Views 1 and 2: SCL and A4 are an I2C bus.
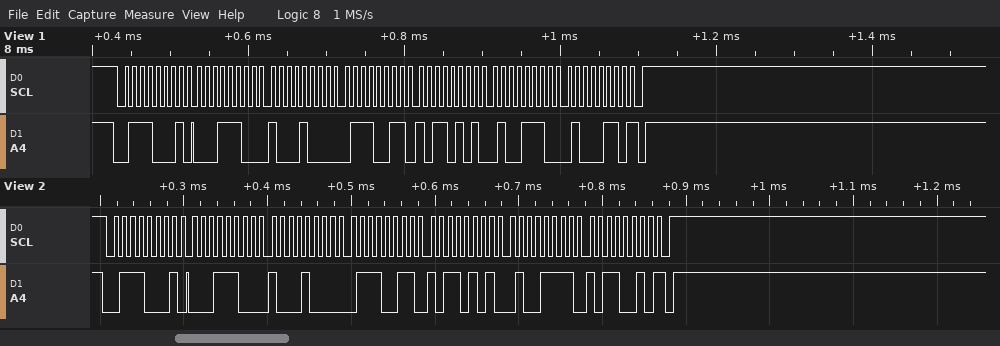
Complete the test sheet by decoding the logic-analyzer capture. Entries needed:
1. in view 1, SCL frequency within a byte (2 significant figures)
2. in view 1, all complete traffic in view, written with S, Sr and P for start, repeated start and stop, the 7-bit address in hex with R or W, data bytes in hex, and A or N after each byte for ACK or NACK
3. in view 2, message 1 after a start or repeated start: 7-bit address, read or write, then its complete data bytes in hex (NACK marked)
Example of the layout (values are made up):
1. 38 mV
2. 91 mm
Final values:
1. 100 kHz
2. S 38R A 1C A 88 A 73 A B5 A 4E A 46 N P
3. 0x38 read: 1C 88 73 B5 4F B2 NACK
